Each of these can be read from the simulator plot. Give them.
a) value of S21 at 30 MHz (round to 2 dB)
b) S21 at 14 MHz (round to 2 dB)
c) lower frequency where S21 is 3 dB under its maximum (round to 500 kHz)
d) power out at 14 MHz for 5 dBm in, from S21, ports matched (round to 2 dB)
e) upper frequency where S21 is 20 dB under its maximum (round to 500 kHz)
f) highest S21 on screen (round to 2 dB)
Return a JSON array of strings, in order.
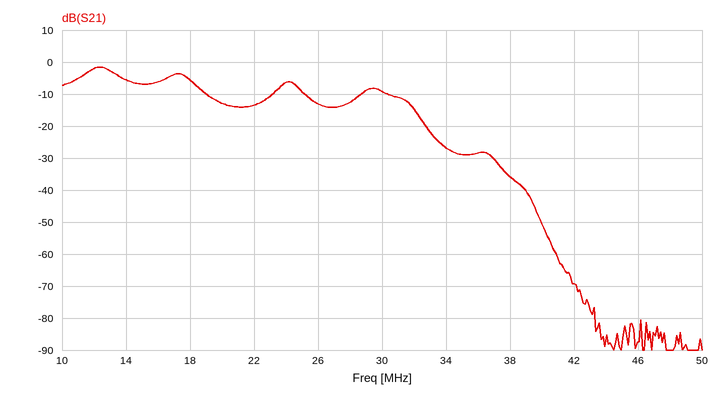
["-10 dB", "-6 dB", "11.0 MHz", "0 dBm", "33.0 MHz", "-2 dB"]
